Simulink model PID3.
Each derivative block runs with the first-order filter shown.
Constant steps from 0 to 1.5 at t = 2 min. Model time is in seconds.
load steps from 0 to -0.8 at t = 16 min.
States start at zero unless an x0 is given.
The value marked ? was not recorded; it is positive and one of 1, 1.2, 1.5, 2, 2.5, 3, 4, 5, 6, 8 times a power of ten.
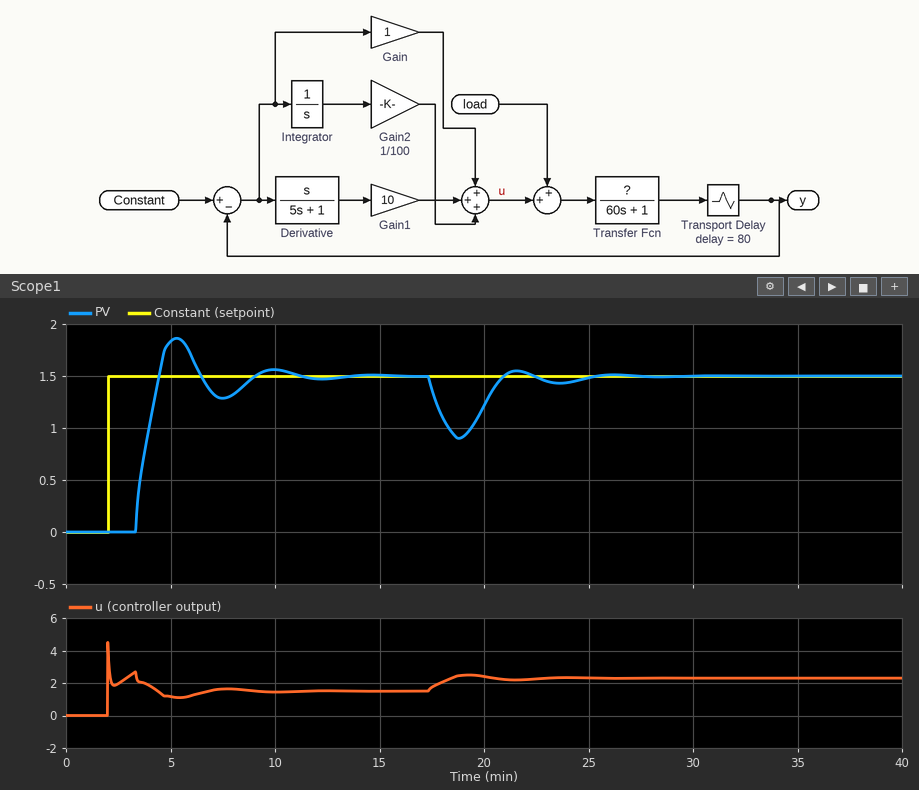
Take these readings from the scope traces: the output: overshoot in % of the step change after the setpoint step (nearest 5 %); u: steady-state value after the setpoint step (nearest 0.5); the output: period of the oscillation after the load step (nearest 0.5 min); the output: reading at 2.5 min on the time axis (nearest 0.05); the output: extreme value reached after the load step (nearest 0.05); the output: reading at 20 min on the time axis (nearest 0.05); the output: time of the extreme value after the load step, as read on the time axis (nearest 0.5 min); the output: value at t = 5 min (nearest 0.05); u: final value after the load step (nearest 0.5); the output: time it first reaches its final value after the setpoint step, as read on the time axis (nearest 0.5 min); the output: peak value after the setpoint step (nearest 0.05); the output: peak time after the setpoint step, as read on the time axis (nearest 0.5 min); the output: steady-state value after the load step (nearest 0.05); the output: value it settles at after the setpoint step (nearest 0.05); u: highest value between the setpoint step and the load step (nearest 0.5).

25 %
1.5
5.0 min
0.00
0.90
1.20
19.0 min
1.85
2.5
4.5 min
1.85
5.5 min
1.50
1.50
4.5
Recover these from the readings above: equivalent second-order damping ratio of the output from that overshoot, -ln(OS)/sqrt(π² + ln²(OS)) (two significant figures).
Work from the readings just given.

0.40
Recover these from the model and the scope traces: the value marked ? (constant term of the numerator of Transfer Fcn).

1
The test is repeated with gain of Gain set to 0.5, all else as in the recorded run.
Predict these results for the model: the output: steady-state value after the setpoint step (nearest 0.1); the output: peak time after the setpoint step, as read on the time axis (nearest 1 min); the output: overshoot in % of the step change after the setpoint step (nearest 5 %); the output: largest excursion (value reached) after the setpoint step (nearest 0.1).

1.5
7 min
20 %
1.8
